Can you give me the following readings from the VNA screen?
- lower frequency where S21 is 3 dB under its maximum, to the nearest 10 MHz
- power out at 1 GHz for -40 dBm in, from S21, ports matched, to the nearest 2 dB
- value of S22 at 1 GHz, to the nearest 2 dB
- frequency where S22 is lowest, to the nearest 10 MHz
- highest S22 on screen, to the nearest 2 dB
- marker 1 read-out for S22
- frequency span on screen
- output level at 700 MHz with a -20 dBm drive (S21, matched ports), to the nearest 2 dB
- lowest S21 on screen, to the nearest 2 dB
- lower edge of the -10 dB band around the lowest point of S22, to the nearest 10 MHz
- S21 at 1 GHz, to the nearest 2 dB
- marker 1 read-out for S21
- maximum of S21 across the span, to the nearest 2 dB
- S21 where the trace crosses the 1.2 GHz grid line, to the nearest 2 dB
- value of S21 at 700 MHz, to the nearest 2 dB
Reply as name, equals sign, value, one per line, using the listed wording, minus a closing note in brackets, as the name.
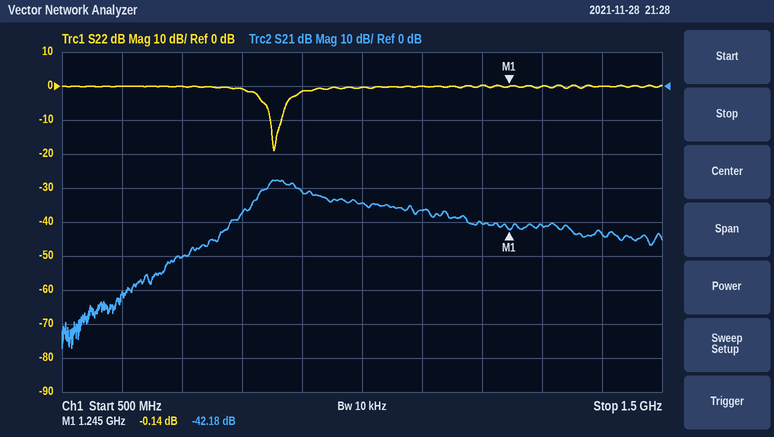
lower frequency where S21 is 3 dB under its maximum, to the nearest 10 MHz = 830 MHz
power out at 1 GHz for -40 dBm in, from S21, ports matched, to the nearest 2 dB = -74 dBm
value of S22 at 1 GHz, to the nearest 2 dB = 0 dB
frequency where S22 is lowest, to the nearest 10 MHz = 850 MHz
highest S22 on screen, to the nearest 2 dB = 0 dB
marker 1 read-out for S22 = -0.14 dB
frequency span on screen = 1 GHz
output level at 700 MHz with a -20 dBm drive (S21, matched ports), to the nearest 2 dB = -70 dBm
lowest S21 on screen, to the nearest 2 dB = -78 dB
lower edge of the -10 dB band around the lowest point of S22, to the nearest 10 MHz = 850 MHz
S21 at 1 GHz, to the nearest 2 dB = -34 dB
marker 1 read-out for S21 = -42.18 dB
maximum of S21 across the span, to the nearest 2 dB = -28 dB
S21 where the trace crosses the 1.2 GHz grid line, to the nearest 2 dB = -40 dB
value of S21 at 700 MHz, to the nearest 2 dB = -50 dB
